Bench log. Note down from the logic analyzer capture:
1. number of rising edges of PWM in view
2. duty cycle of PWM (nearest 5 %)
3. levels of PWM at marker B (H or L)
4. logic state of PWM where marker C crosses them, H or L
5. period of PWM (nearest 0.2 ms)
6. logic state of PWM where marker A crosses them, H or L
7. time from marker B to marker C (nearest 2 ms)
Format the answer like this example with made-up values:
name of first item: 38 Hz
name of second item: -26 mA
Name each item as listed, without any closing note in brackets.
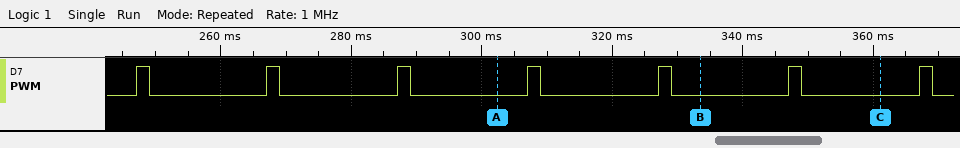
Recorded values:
number of rising edges of PWM in view: 7
duty cycle of PWM: 10 %
levels of PWM at marker B: PWM=L
logic state of PWM where marker C crosses them, H or L: PWM=L
period of PWM: 20 ms
logic state of PWM where marker A crosses them, H or L: PWM=L
time from marker B to marker C: 28 ms
